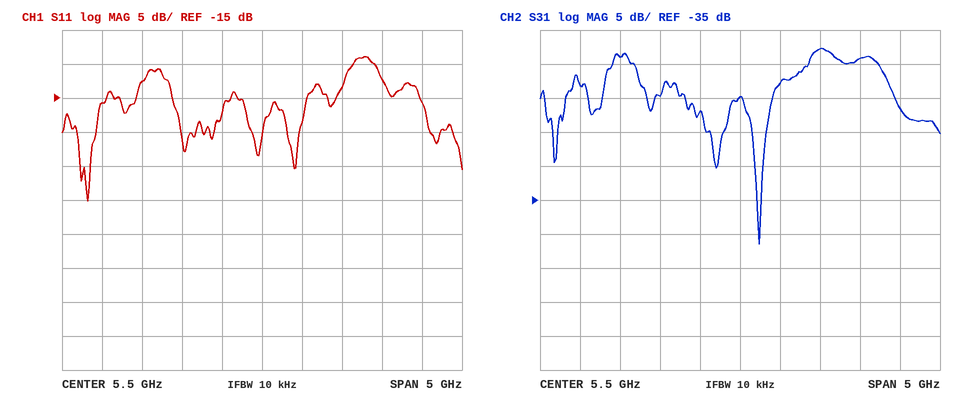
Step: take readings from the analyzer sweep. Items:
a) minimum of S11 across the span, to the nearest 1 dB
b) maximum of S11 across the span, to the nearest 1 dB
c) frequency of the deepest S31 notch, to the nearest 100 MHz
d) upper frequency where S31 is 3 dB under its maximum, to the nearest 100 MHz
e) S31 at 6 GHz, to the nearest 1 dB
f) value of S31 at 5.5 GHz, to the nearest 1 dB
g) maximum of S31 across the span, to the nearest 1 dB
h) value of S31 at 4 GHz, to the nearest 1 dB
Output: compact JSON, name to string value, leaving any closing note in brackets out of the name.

{"minimum of S11 across the span, to the nearest 1 dB": "-30 dB", "maximum of S11 across the span, to the nearest 1 dB": "-9 dB", "frequency of the deepest S31 notch, to the nearest 100 MHz": "5.7 GHz", "upper frequency where S31 is 3 dB under its maximum, to the nearest 100 MHz": "7.3 GHz", "S31 at 6 GHz, to the nearest 1 dB": "-18 dB", "value of S31 at 5.5 GHz, to the nearest 1 dB": "-20 dB", "maximum of S31 across the span, to the nearest 1 dB": "-13 dB", "value of S31 at 4 GHz, to the nearest 1 dB": "-14 dB"}
